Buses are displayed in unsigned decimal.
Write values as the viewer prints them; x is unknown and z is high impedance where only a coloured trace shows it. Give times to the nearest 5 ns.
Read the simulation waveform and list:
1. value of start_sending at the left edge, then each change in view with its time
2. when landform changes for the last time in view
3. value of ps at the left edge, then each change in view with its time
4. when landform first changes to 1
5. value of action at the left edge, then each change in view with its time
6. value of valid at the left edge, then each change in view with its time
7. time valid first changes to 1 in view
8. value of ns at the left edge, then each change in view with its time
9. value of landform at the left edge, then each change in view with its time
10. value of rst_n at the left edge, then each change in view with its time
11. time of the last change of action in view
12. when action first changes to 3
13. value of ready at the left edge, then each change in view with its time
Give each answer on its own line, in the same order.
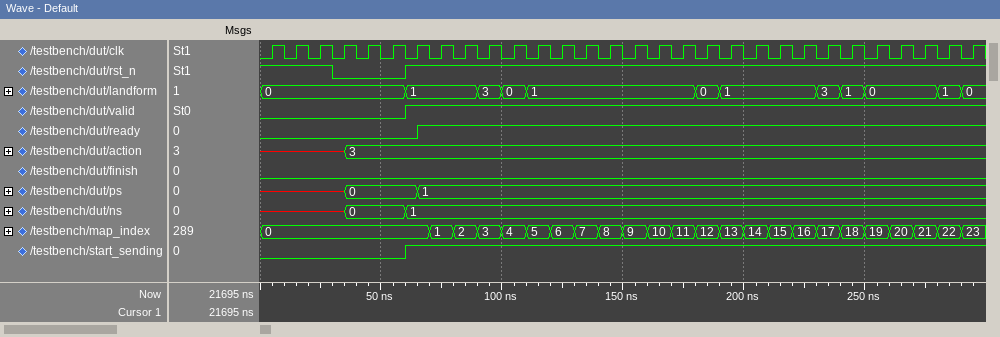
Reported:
0, 1 at 60 ns
290 ns
x, 0 at 35 ns, 1 at 65 ns
60 ns
x, 3 at 35 ns
0, 1 at 60 ns
60 ns
x, 0 at 35 ns, 1 at 60 ns
0, 1 at 60 ns, 3 at 90 ns, 0 at 100 ns, 1 at 110 ns, 0 at 180 ns, 1 at 190 ns, 3 at 230 ns, 1 at 240 ns, 0 at 250 ns, 1 at 280 ns, 0 at 290 ns
1, 0 at 30 ns, 1 at 60 ns
35 ns
35 ns
0, 1 at 65 ns
